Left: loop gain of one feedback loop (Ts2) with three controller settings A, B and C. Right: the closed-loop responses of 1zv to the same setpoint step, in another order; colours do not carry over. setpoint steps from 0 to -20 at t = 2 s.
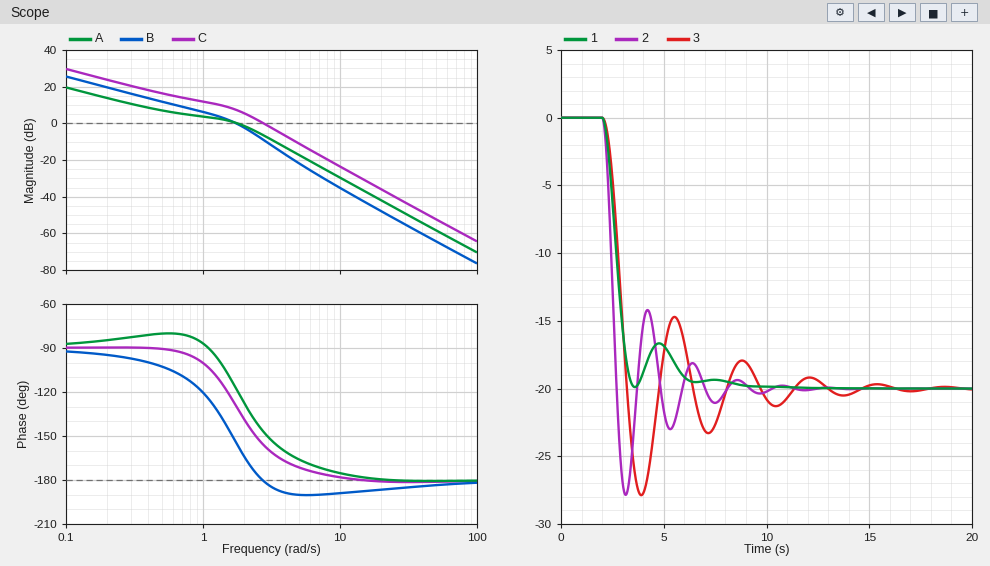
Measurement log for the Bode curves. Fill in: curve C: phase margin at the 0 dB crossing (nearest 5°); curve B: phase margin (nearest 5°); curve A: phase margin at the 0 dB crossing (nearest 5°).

25°
25°
60°
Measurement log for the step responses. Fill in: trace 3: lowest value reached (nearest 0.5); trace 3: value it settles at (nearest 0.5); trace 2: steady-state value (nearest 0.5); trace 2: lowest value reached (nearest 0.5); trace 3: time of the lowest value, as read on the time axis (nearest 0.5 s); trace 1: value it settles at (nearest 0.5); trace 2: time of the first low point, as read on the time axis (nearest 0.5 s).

-28.0
-20.0
-20.0
-28.0
4.0 s
-20.0
3.0 s
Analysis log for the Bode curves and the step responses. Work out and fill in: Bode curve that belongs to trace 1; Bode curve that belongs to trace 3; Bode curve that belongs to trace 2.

A
B
C
